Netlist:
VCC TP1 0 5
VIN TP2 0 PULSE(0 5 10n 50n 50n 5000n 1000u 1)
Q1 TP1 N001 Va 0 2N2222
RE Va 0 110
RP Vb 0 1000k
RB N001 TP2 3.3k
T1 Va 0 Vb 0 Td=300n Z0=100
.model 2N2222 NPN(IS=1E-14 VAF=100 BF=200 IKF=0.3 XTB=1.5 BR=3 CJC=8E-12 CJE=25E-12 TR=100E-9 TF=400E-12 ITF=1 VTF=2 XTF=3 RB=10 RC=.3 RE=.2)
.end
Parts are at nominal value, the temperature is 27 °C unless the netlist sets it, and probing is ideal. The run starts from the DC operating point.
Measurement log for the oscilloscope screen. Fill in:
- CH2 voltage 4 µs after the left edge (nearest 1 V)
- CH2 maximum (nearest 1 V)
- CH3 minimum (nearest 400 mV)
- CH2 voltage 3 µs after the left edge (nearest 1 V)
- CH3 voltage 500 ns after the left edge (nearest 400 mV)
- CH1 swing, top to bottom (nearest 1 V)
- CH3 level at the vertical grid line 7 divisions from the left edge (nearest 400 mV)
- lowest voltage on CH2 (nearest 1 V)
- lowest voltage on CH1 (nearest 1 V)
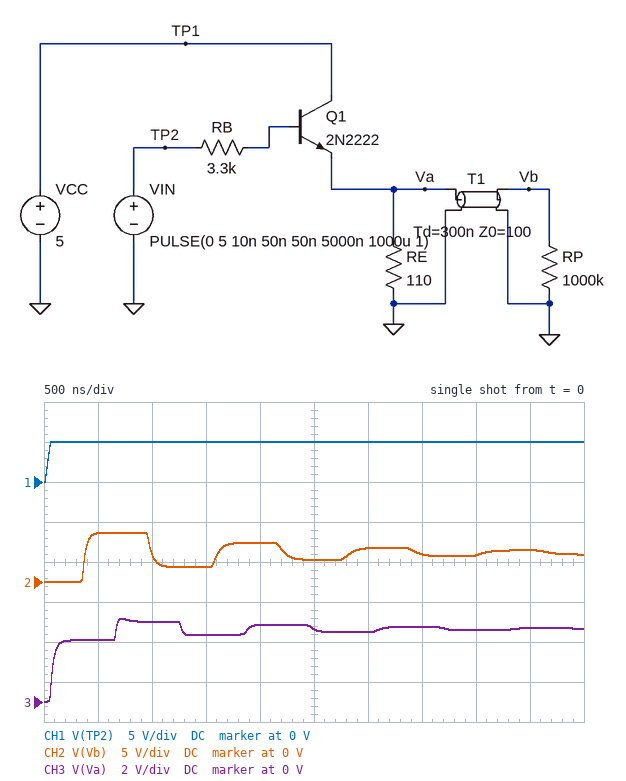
3 V
6 V
0 V
4 V
3.2 V
5 V
3.6 V
0 V
0 V
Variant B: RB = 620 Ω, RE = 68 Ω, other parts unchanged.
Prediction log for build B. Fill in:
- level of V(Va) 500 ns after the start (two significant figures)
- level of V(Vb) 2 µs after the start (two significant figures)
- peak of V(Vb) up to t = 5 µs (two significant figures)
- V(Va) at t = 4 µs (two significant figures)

3.8 V
7.0 V
7.6 V
3.9 V
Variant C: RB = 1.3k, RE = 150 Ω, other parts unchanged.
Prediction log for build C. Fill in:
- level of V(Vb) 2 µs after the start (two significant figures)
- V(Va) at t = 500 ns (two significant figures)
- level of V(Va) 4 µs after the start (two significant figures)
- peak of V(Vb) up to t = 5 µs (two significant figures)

6.2 V
3.7 V
4.0 V
7.5 V
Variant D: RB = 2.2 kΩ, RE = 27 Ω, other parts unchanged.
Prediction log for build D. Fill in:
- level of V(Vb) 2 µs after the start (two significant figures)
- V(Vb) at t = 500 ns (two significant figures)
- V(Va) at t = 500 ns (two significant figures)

4.2 V
4.9 V
2.5 V
